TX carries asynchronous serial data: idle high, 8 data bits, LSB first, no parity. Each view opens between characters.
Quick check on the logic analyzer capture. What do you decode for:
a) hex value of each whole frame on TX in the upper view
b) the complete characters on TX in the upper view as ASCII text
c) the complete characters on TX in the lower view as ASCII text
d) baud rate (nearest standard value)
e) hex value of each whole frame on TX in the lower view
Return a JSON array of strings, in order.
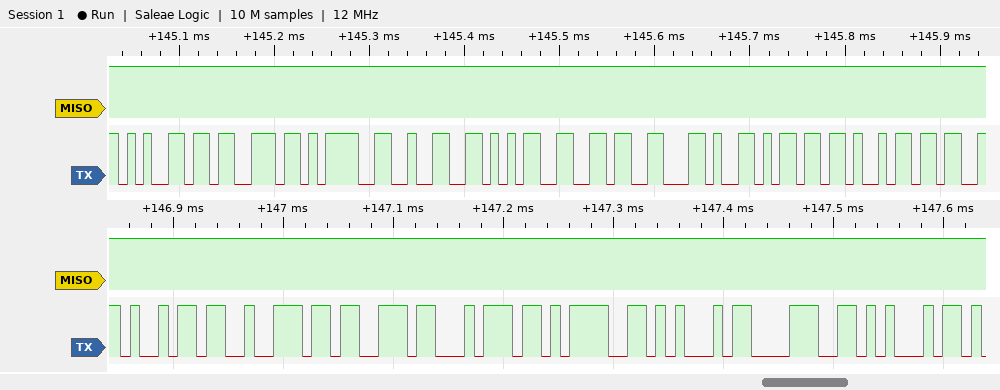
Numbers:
["65, 73, 3D, 32, 35, 36, 2C, 6D, 69", "\"es=256,mi\"", "\"irst=E8E\"", "115200 baud", "69, 72, 73, 74, 3D, 45, 38, 45"]
